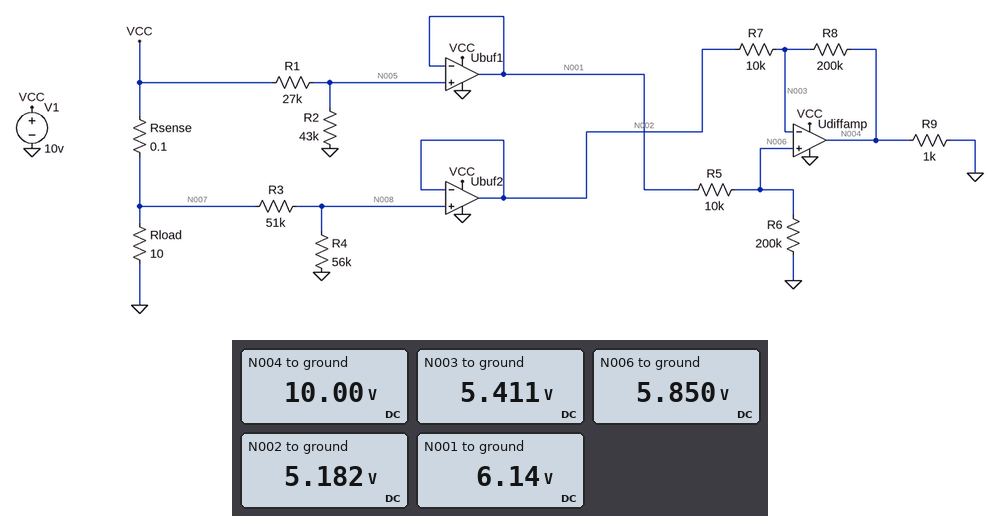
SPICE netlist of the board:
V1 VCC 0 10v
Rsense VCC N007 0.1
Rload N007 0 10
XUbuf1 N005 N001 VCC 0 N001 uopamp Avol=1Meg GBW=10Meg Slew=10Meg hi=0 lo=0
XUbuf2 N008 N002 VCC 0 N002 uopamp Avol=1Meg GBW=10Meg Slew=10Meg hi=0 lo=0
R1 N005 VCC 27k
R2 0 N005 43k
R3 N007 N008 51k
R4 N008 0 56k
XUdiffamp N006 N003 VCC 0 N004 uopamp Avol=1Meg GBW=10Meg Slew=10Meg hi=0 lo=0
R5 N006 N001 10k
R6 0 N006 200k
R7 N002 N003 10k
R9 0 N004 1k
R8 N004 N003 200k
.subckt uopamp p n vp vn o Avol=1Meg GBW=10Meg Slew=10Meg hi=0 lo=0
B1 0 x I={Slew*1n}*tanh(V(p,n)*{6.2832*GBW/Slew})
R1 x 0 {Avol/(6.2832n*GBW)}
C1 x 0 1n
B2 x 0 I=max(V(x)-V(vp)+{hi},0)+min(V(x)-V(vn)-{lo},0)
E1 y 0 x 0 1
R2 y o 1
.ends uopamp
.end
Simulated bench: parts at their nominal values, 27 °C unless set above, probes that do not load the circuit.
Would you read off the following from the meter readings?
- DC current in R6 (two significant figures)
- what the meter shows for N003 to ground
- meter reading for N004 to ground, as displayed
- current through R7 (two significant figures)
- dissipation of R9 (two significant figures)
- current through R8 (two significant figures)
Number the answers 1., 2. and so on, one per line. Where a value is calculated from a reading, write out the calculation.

1. (5.85 V) / 200 kΩ = 29 µA
2. 5.411 V
3. 10.00 V
4. (5.411 V - 5.182 V) / 10 kΩ = 23 µA
5. (10 V)^2 / 1 kΩ = 100 mW
6. (10 V - 5.411 V) / 200 kΩ = 23 µA
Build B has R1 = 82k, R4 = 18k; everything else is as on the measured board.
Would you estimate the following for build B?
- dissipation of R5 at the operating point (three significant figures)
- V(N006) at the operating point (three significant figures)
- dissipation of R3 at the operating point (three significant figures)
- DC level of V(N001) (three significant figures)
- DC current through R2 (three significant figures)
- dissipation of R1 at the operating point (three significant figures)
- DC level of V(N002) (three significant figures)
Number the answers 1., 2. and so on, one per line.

1. 2.68 µW
2. 3.28 V
3. 1.05 mW
4. 3.44 V
5. 80.0 µA
6. 525 µW
7. 2.58 V
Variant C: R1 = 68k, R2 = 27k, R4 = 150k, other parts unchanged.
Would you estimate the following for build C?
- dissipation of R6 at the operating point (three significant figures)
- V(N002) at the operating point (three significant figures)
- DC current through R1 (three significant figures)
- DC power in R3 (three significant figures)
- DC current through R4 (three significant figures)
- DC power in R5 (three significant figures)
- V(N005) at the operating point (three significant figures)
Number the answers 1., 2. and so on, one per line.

1. 36.6 µW
2. 7.39 V
3. 105 µA
4. 124 µW
5. 49.3 µA
6. 1.83 µW
7. 2.84 V
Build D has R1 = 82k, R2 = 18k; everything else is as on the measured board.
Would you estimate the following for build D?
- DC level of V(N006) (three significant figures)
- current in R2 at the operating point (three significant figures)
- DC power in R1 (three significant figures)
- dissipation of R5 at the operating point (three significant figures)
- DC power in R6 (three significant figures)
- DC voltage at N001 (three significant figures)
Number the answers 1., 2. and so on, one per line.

1. 1.71 V
2. 100 µA
3. 820 µW
4. 735 nW
5. 14.7 µW
6. 1.80 V
